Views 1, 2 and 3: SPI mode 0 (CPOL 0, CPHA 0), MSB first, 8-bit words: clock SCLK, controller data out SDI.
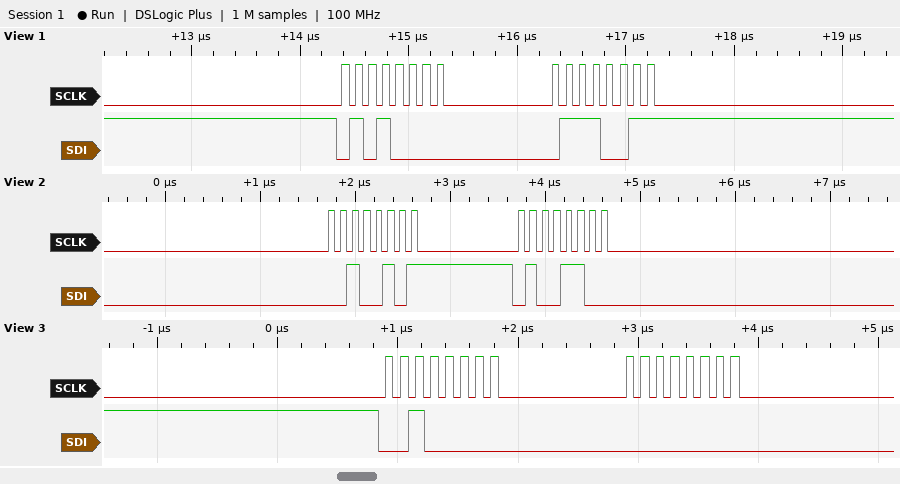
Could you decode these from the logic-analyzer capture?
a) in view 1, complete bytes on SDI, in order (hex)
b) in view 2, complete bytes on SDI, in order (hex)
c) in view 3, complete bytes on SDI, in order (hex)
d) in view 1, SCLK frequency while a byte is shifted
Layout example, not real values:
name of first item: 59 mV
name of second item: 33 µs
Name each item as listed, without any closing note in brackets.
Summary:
in view 1, complete bytes on SDI, in order: 50 73
in view 2, complete bytes on SDI, in order: 25 4C
in view 3, complete bytes on SDI, in order: 20 00
in view 1, SCLK frequency while a byte is shifted: 8 MHz
